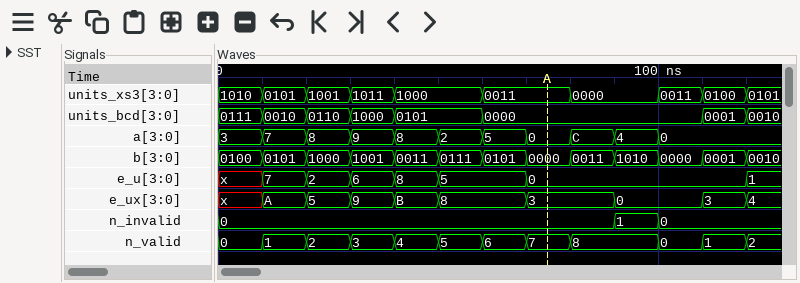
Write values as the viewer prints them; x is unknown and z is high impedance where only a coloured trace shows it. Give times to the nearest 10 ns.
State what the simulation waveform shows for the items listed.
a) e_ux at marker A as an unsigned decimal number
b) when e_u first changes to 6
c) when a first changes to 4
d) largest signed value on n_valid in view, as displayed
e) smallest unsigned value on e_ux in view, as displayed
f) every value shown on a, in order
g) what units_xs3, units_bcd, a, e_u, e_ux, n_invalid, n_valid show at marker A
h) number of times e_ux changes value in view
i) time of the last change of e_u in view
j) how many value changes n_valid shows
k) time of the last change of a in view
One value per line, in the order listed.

3
30 ns
90 ns
8
0
3, 7, 8, 9, 8, 2, 5, 0, C, 4, 0
units_xs3=0011, units_bcd=0000, a=0, e_u=0, e_ux=3, n_invalid=0, n_valid=7
9
120 ns
11
100 ns
